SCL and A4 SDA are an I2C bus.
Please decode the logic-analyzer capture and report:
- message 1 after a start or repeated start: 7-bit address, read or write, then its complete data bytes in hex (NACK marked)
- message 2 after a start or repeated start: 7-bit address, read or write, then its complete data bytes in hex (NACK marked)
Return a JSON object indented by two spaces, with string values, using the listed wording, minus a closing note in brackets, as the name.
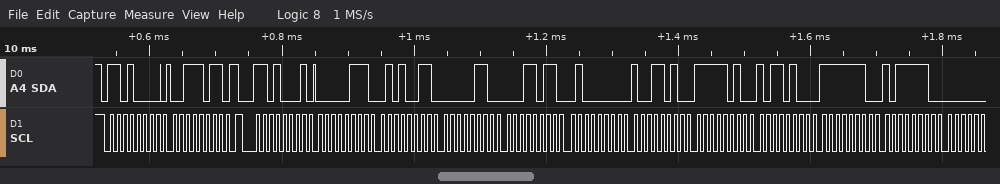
{
  "message 1 after a start or repeated start: 7-bit address, read or write, then its complete data bytes in hex": "0x68 write: 3B",
  "message 2 after a start or repeated start: 7-bit address, read or write, then its complete data bytes in hex": "0x68 read: 07 53 06 1B 40 9A FA B4 FE BE"
}
